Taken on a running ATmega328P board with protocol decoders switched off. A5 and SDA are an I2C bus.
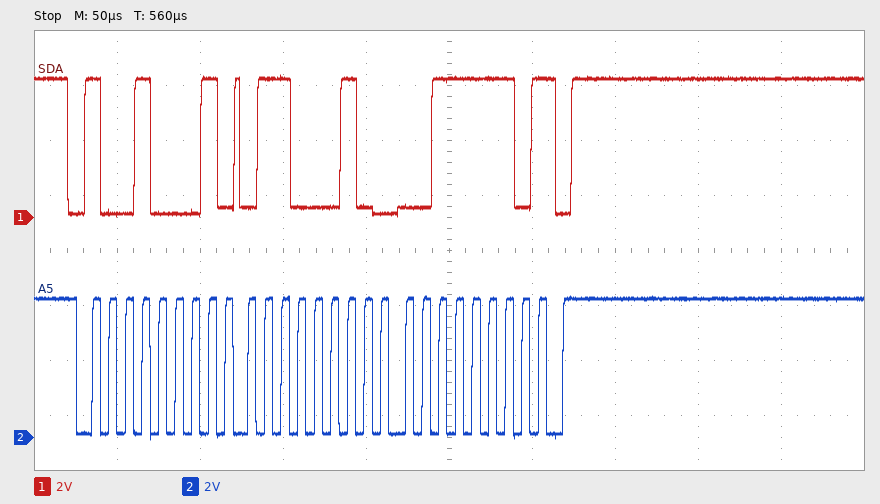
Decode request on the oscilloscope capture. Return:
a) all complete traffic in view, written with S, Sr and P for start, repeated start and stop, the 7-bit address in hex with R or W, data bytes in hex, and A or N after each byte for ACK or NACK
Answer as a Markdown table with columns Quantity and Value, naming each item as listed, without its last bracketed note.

| Quantity | Value |
|---|---|
| all complete traffic in view, written with S, Sr and P for start, repeated start and stop, the 7-bit address in hex with R or W, data bytes in hex, and A or N after each byte for ACK or NACK | S 48R A 62 A 3E N P |
